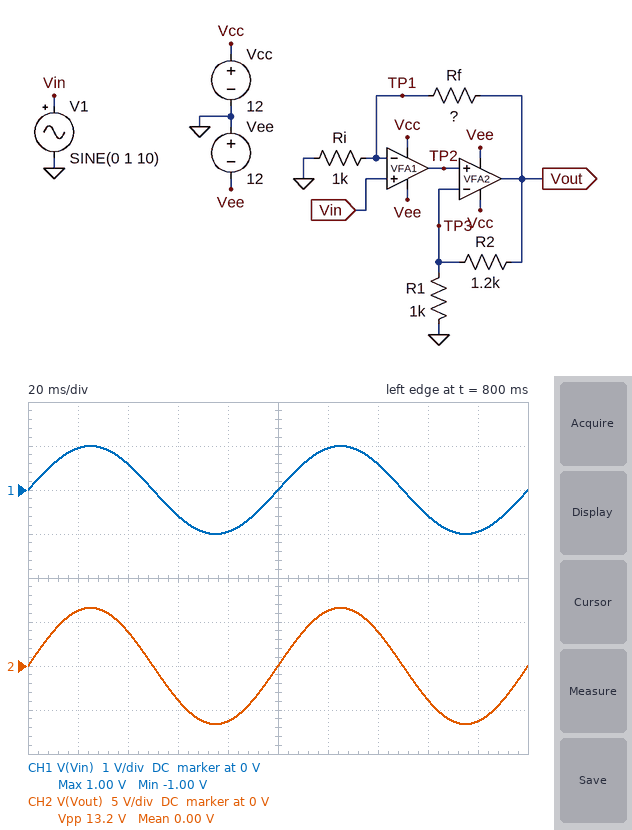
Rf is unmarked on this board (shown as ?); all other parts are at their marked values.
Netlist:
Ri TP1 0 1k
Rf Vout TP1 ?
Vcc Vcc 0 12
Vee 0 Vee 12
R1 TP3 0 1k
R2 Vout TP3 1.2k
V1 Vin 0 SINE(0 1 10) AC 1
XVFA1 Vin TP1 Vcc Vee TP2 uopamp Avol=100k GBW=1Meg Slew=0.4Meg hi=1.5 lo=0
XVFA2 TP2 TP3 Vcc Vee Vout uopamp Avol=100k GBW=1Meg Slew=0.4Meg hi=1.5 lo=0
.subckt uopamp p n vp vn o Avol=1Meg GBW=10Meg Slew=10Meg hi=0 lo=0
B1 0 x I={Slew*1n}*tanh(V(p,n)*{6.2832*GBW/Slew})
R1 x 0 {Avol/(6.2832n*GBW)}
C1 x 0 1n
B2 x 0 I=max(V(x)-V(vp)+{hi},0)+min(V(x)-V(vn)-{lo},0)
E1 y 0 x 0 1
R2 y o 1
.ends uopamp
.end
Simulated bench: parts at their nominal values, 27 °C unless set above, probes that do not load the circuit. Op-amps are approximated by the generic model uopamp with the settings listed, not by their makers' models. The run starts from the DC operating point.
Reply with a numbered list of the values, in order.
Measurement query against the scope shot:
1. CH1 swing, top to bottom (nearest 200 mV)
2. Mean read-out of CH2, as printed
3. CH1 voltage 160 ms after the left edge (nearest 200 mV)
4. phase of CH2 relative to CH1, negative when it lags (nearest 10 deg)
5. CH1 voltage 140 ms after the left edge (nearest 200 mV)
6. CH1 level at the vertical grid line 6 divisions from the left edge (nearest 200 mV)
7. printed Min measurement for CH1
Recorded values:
1. 2.0 V
2. 0.00 V
3. -600 mV
4. 0 deg
5. 600 mV
6. 1.0 V
7. -1.00 V
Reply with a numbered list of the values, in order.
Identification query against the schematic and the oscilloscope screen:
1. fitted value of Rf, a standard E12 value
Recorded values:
1. 5.6 kΩ
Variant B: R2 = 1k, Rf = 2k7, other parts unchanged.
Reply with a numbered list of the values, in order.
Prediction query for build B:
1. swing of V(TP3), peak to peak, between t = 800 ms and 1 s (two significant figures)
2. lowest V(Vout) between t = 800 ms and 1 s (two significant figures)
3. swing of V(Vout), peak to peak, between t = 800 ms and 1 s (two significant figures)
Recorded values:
1. 3.7 V
2. -3.7 V
3. 7.4 V
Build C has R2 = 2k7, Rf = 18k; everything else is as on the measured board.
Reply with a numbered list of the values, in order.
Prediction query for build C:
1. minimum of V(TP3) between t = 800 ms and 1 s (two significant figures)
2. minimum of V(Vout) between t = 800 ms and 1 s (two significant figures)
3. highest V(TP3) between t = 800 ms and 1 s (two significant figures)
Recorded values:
1. -3.2 V
2. -12 V
3. 2.8 V
